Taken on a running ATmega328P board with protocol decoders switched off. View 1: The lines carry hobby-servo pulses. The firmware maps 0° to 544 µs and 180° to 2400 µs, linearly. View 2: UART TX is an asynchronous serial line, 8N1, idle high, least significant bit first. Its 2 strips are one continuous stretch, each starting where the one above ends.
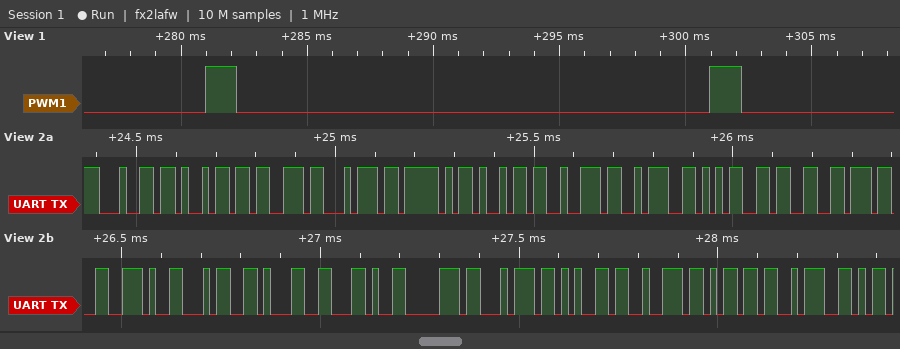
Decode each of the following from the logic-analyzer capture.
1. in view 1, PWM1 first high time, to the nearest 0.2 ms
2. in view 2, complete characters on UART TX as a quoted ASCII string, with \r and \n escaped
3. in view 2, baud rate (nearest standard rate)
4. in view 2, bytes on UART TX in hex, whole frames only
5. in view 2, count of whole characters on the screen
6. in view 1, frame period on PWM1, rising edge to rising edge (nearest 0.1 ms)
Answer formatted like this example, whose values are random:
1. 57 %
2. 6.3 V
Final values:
1. 1.2 ms
2. "dist_ir:537.41,pterm:"
3. 57600 baud
4. 0x64 0x69 0x73 0x74 0x5F 0x69 0x72 0x3A 0x35 0x33 0x37 0x2E 0x34 0x31 0x2C 0x70 0x74 0x65 0x72 0x6D 0x3A
5. 21
6. 20.0 ms
